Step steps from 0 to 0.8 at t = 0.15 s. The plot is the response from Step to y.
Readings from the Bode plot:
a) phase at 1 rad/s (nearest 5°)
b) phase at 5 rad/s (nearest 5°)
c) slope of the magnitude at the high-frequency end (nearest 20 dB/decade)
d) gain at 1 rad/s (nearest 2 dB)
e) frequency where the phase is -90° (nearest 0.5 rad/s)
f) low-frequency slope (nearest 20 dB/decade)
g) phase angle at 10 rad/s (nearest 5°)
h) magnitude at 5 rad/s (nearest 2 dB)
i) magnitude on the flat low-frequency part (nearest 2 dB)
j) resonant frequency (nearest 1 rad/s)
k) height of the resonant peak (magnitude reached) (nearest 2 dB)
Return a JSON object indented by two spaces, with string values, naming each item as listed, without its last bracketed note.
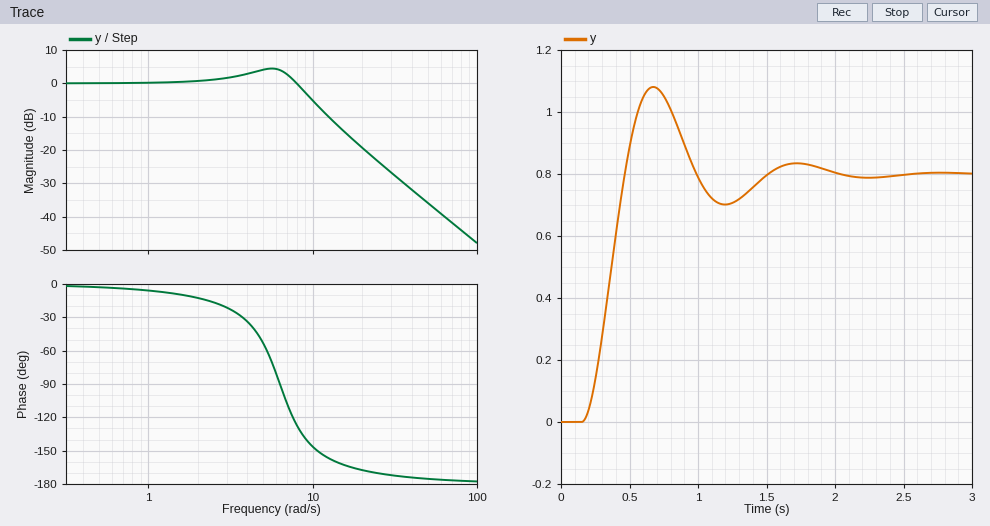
{
  "phase at 1 rad/s": "-5°",
  "phase at 5 rad/s": "-55°",
  "slope of the magnitude at the high-frequency end": "-40 dB/decade",
  "gain at 1 rad/s": "0 dB",
  "frequency where the phase is -90°": "6.5 rad/s",
  "low-frequency slope": "0 dB/decade",
  "phase angle at 10 rad/s": "-145°",
  "magnitude at 5 rad/s": "4 dB",
  "magnitude on the flat low-frequency part": "0 dB",
  "resonant frequency": "6 rad/s",
  "height of the resonant peak (magnitude reached)": "4 dB"
}
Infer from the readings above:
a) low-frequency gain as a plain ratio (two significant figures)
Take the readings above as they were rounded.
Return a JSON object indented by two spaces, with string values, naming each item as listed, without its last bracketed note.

{
  "low-frequency gain as a plain ratio": "1.0"
}
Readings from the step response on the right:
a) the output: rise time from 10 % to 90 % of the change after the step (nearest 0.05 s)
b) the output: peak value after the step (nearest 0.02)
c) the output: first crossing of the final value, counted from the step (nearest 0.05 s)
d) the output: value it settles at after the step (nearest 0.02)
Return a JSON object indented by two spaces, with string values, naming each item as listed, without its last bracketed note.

{
  "the output: rise time from 10 % to 90 % of the change after the step": "0.20 s",
  "the output: peak value after the step": "1.08",
  "the output: first crossing of the final value, counted from the step": "0.30 s",
  "the output: value it settles at after the step": "0.80"
}
